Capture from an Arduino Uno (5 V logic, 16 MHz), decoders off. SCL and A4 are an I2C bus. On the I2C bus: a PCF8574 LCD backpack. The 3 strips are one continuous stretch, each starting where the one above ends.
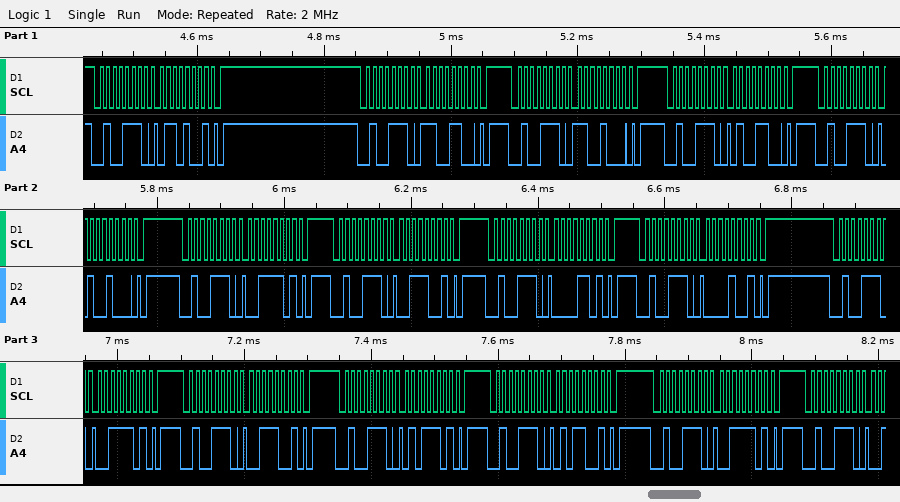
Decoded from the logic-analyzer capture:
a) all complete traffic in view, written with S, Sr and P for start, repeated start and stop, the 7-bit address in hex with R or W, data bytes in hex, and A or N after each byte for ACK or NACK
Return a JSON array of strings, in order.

["S 27W A 69 A P S 27W A CC A P S 27W A C8 A P S 27W A 4C A P S 27W A 48 A P S 27W A 3D A P S 27W A 39 A P S 27W A 0D A P S 27W A 09 A P S 27W A 3D A P S 27W A 39 A P S 27W A 5D A P S 27W A 59 A P S 27W A 3D A P S 27W A"]
